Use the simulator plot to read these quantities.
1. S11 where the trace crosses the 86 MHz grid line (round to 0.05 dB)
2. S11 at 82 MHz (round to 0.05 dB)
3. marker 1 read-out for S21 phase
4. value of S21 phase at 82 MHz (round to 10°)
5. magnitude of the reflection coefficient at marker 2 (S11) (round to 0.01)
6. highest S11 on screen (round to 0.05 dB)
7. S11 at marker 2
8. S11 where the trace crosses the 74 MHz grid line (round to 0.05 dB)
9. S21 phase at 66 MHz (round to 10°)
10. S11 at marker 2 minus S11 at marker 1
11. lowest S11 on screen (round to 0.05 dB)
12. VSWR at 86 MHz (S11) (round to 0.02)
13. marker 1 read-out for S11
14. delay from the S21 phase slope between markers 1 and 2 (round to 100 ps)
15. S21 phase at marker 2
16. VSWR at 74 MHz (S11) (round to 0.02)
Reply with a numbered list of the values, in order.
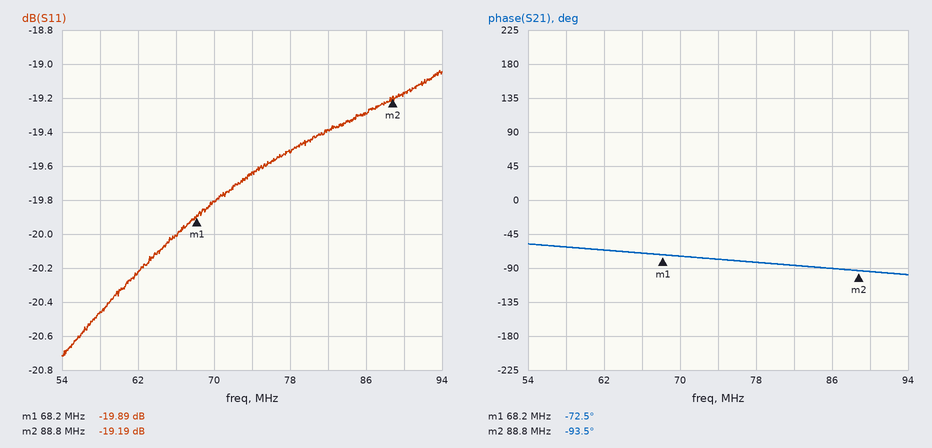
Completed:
1. -19.30 dB
2. -19.40 dB
3. -72.5°
4. -90°
5. 0.11
6. -19.05 dB
7. -19.19 dB
8. -19.65 dB
9. -70°
10. 0.70 dB
11. -20.70 dB
12. 1.24
13. -19.89 dB
14. 2.8 ns
15. -93.5°
16. 1.24
